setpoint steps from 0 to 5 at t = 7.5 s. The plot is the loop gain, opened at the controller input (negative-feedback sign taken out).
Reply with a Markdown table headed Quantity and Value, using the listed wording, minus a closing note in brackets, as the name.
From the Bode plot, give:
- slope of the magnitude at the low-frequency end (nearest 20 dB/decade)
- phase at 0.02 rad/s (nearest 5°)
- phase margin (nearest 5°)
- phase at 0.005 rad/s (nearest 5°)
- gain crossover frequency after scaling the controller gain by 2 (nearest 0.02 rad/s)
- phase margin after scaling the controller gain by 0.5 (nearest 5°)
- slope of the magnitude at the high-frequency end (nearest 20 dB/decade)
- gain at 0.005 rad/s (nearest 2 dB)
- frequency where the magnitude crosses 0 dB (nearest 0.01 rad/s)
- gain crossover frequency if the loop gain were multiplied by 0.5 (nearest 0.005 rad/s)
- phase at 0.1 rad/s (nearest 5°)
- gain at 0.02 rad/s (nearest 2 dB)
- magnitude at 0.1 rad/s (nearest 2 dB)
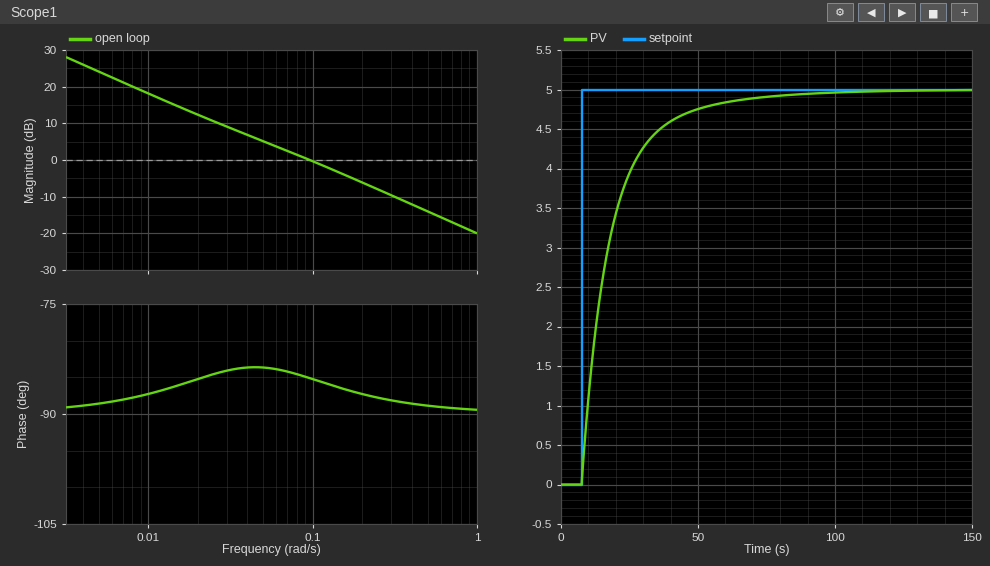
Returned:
| Quantity | Value |
|---|---|
| slope of the magnitude at the low-frequency end | -20 dB/decade |
| phase at 0.02 rad/s | -85° |
| phase margin | 95° |
| phase at 0.005 rad/s | -90° |
| gain crossover frequency after scaling the controller gain by 2 | 0.20 rad/s |
| phase margin after scaling the controller gain by 0.5 | 95° |
| slope of the magnitude at the high-frequency end | -20 dB/decade |
| gain at 0.005 rad/s | 24 dB |
| frequency where the magnitude crosses 0 dB | 0.10 rad/s |
| gain crossover frequency if the loop gain were multiplied by 0.5 | 0.045 rad/s |
| phase at 0.1 rad/s | -85° |
| gain at 0.02 rad/s | 12 dB |
| magnitude at 0.1 rad/s | 0 dB |
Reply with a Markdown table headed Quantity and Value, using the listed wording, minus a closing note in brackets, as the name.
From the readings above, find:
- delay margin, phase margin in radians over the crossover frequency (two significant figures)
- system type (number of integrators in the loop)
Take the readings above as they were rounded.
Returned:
| Quantity | Value |
|---|---|
| delay margin, phase margin in radians over the crossover frequency | 17 s |
| system type | 1 |
